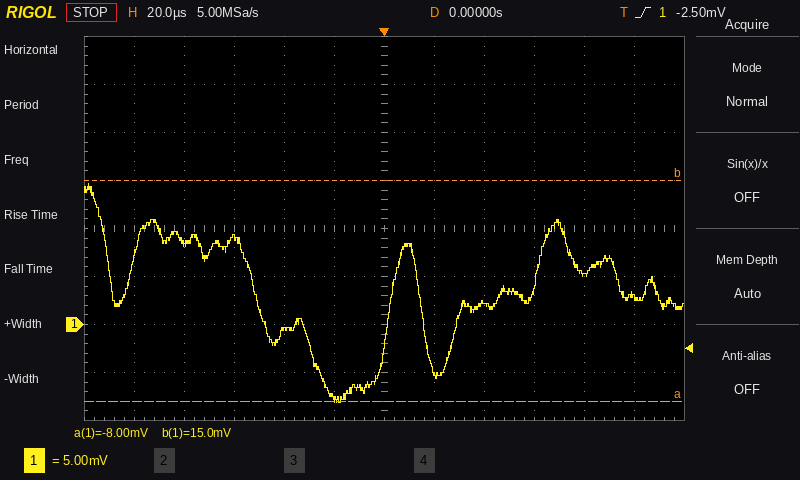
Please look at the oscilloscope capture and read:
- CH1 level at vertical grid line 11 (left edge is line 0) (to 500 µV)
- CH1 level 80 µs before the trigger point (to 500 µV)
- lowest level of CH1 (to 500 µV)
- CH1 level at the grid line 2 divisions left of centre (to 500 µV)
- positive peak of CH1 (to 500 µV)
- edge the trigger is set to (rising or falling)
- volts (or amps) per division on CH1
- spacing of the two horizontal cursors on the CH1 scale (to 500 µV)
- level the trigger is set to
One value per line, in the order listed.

3.0 mV
8.5 mV
-8.0 mV
-500 µV
14.5 mV
rising
5 mV
23.0 mV
-2.50 mV
